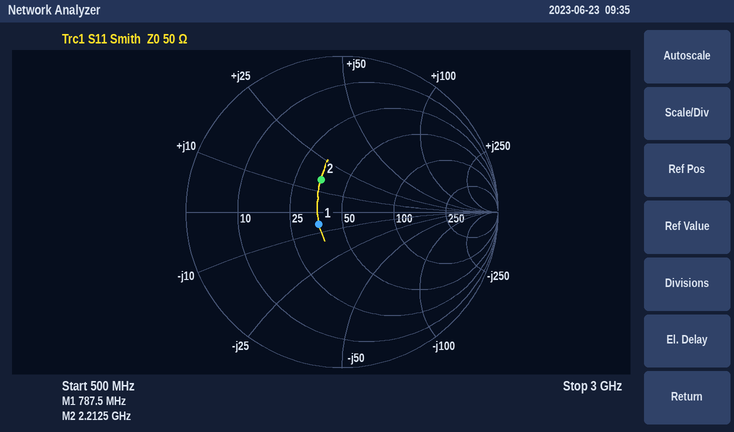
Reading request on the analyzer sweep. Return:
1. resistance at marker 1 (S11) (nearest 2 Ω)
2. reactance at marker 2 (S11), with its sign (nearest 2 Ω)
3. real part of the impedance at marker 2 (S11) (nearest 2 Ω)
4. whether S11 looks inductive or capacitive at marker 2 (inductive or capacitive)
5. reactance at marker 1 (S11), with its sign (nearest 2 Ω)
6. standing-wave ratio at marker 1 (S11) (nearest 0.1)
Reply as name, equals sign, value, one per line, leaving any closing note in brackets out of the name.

resistance at marker 1 (S11) = 36 Ω
reactance at marker 2 (S11), with its sign = +16 Ω
real part of the impedance at marker 2 (S11) = 36 Ω
whether S11 looks inductive or capacitive at marker 2 = inductive
reactance at marker 1 (S11), with its sign = -6 Ω
standing-wave ratio at marker 1 (S11) = 1.4
